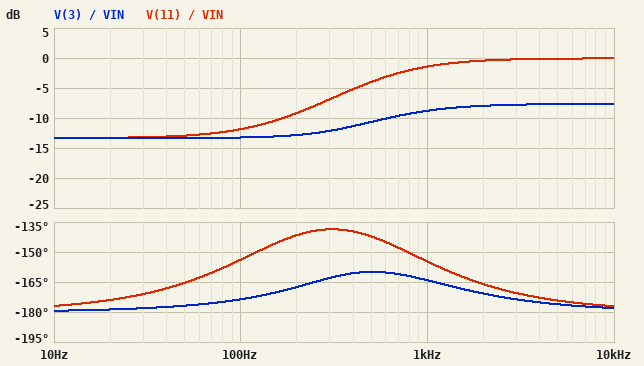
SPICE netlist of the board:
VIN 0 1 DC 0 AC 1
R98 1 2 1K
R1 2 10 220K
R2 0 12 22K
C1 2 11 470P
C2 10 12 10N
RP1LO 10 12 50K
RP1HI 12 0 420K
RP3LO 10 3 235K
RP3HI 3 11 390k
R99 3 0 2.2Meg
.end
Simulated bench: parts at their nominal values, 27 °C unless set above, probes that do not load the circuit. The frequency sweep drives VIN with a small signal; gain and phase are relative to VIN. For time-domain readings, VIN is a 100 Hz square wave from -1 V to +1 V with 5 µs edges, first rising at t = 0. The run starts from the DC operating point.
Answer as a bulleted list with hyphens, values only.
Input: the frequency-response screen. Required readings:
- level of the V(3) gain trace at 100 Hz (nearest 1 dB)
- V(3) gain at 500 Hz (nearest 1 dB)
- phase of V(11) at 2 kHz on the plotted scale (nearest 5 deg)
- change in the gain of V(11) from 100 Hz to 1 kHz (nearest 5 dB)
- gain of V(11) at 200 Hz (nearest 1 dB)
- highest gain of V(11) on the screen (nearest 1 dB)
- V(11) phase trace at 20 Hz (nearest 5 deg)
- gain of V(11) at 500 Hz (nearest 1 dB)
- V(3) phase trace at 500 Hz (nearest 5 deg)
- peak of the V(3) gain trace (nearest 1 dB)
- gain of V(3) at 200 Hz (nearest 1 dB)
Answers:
- -13 dB
- -11 dB
- -165 deg
- 10 dB
- -9 dB
- 0 dB
- -175 deg
- -4 dB
- -160 deg
- -8 dB
- -13 dB
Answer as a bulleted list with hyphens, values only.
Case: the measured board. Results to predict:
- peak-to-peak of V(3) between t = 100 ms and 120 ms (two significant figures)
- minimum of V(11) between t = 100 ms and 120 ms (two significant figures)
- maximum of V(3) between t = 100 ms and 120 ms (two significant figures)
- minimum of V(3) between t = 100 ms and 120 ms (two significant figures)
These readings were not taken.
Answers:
- 1.2 V
- -1.8 V
- 610 mV
- -610 mV
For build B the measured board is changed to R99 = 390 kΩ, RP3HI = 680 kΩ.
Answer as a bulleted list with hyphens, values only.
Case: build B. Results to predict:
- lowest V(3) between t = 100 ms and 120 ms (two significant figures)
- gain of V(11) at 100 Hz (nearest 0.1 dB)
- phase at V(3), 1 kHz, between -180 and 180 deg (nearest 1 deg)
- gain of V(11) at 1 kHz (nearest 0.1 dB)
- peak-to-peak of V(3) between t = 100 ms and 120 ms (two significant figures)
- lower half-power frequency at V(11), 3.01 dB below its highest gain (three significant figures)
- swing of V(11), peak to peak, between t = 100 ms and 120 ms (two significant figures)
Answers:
- -310 mV
- -11.8 dB
- -172 deg
- -0.8 dB
- 620 mV
- 438 Hz
- 3.7 V
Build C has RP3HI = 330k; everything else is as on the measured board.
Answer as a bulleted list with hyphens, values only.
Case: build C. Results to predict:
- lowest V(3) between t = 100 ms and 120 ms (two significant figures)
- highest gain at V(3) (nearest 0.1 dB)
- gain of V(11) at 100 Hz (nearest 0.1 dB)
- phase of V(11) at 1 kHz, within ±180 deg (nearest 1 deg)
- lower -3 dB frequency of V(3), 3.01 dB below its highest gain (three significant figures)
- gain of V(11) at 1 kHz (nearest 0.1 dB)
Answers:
- -680 mV
- -6.9 dB
- -12.2 dB
- -153 deg
- 598 Hz
- -1.7 dB
